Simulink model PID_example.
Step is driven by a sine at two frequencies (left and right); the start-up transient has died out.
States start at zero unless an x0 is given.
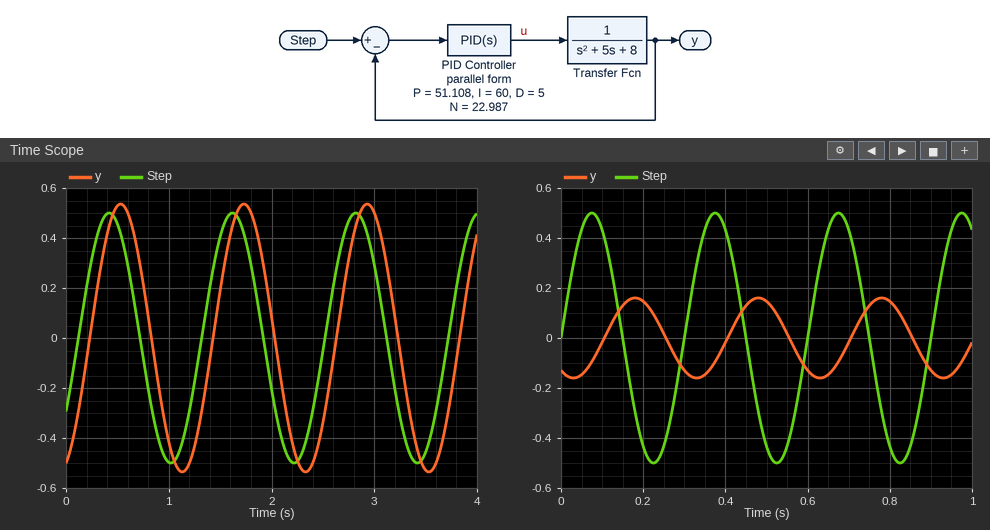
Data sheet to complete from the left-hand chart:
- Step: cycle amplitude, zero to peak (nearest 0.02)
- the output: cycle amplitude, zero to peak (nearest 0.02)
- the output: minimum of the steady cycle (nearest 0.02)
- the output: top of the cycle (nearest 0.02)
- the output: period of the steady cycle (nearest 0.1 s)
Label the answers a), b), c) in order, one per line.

a) 0.50
b) 0.54
c) -0.54
d) 0.54
e) 1.2 s
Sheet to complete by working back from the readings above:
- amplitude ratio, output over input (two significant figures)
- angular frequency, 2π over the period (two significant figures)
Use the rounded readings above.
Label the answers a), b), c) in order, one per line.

a) 1.1
b) 5.2 rad/s
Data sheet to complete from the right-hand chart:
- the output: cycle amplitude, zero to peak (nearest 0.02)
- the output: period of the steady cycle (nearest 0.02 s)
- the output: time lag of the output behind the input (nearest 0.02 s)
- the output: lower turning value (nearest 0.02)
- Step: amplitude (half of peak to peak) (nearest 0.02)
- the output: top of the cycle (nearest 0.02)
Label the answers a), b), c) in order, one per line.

a) 0.16
b) 0.30 s
c) 0.10 s
d) -0.16
e) 0.50
f) 0.16
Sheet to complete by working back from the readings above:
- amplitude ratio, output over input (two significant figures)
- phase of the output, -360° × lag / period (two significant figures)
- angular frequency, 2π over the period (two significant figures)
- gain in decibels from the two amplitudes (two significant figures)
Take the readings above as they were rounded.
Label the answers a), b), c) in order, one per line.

a) 0.32
b) -120°
c) 21 rad/s
d) -9.9 dB
